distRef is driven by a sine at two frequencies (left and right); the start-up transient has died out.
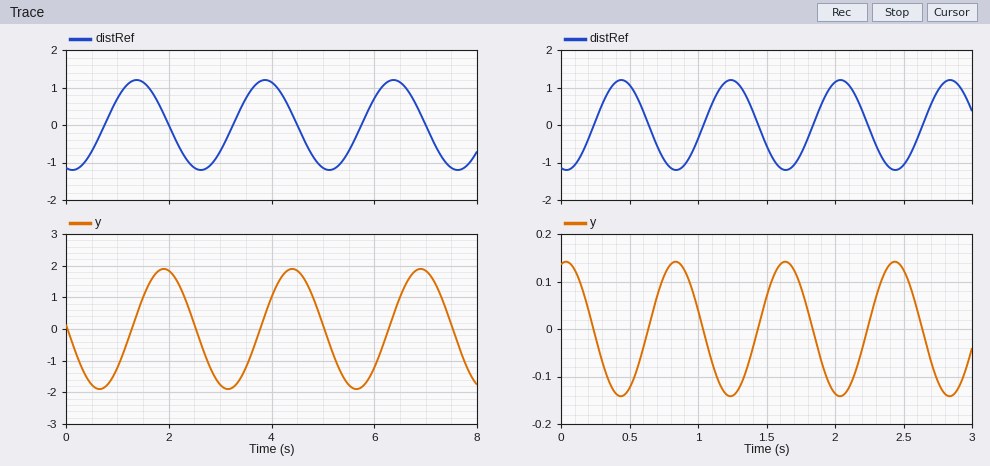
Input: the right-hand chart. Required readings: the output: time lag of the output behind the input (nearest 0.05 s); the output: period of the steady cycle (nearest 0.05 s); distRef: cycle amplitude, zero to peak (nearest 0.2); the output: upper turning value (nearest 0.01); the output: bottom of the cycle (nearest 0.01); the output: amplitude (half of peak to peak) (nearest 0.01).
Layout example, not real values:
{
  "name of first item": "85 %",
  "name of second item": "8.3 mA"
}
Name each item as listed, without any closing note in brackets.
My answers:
{
  "the output: time lag of the output behind the input": "0.40 s",
  "the output: period of the steady cycle": "0.80 s",
  "distRef: cycle amplitude, zero to peak": "1.2",
  "the output: upper turning value": "0.14",
  "the output: bottom of the cycle": "-0.14",
  "the output: amplitude (half of peak to peak)": "0.14"
}
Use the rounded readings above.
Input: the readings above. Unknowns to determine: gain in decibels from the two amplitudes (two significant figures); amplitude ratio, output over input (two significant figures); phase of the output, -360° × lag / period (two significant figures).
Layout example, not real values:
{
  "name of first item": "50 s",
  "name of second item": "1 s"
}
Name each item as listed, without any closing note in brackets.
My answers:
{
  "gain in decibels from the two amplitudes": "-19 dB",
  "amplitude ratio, output over input": "0.12",
  "phase of the output, -360° × lag / period": "-180°"
}
